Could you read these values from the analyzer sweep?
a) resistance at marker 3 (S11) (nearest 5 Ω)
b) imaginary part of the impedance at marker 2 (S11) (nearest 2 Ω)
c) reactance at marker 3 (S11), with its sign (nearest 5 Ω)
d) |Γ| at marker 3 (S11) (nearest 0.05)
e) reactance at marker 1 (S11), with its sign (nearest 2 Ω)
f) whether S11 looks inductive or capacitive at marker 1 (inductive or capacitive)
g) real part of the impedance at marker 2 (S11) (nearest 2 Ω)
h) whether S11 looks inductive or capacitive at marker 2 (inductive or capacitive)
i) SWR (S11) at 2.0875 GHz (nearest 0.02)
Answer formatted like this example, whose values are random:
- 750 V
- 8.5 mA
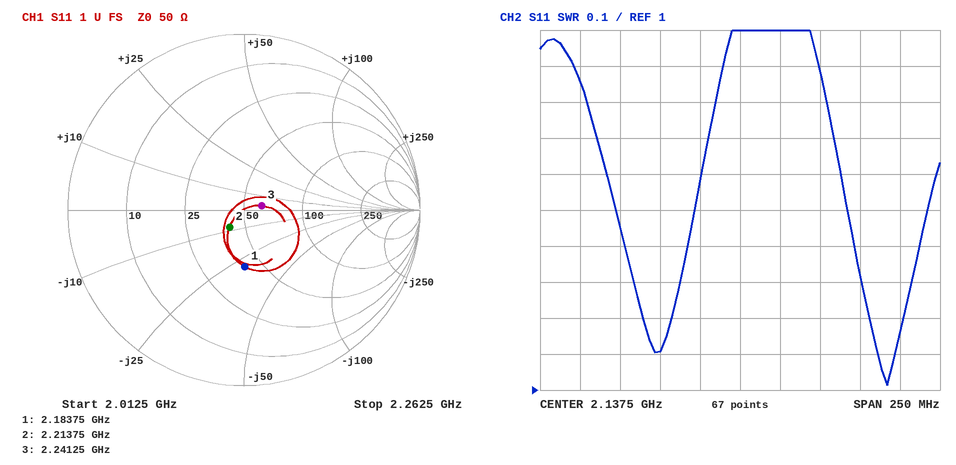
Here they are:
- 60 Ω
- -8 Ω
- +5 Ω
- 0.10
- -30 Ω
- capacitive
- 42 Ω
- capacitive
- 1.10
